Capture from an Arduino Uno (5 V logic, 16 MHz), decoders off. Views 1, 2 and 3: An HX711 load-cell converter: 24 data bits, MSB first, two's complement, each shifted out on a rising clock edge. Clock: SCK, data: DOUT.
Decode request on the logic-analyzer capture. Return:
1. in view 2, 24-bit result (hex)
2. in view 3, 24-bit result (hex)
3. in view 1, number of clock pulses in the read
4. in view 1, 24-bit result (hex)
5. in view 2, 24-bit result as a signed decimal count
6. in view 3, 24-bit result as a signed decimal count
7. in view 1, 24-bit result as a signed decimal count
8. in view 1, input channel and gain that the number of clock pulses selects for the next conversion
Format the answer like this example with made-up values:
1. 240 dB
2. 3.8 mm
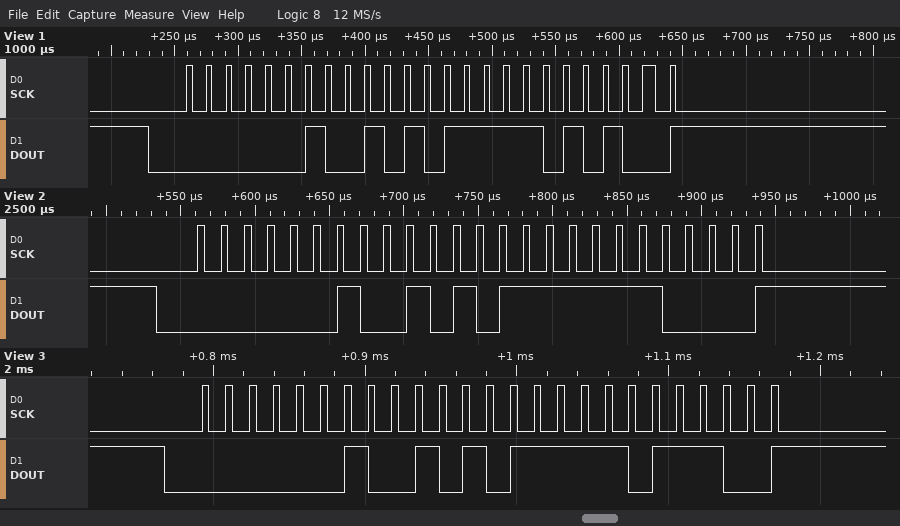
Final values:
1. 0x0257F0
2. 0x0257DC
3. 25
4. 0x0257D4
5. 153584
6. 153564
7. 153556
8. channel A, gain 128
